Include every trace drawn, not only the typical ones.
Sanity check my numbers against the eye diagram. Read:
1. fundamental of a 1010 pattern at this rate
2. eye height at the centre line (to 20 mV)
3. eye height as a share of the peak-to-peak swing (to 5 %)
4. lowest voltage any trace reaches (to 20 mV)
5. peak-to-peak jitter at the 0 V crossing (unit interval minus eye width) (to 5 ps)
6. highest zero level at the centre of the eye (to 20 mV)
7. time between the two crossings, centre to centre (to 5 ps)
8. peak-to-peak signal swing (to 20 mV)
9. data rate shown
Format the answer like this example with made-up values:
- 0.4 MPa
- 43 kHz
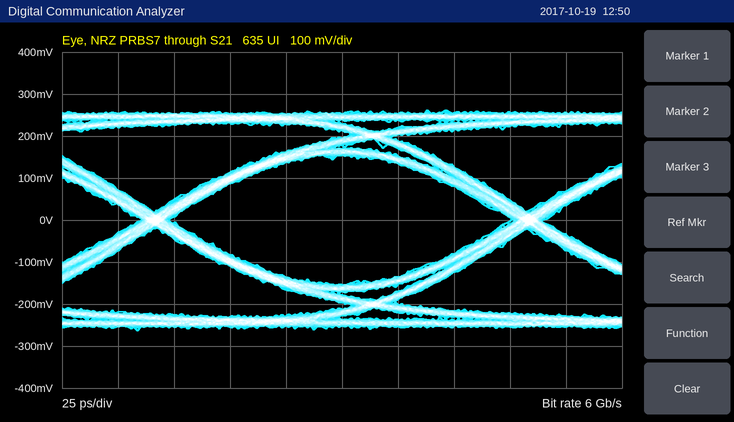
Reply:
- 3 GHz
- 300 mV
- 60 %
- -260 mV
- 15 ps
- -160 mV
- 165 ps
- 520 mV
- 6 Gb/s
